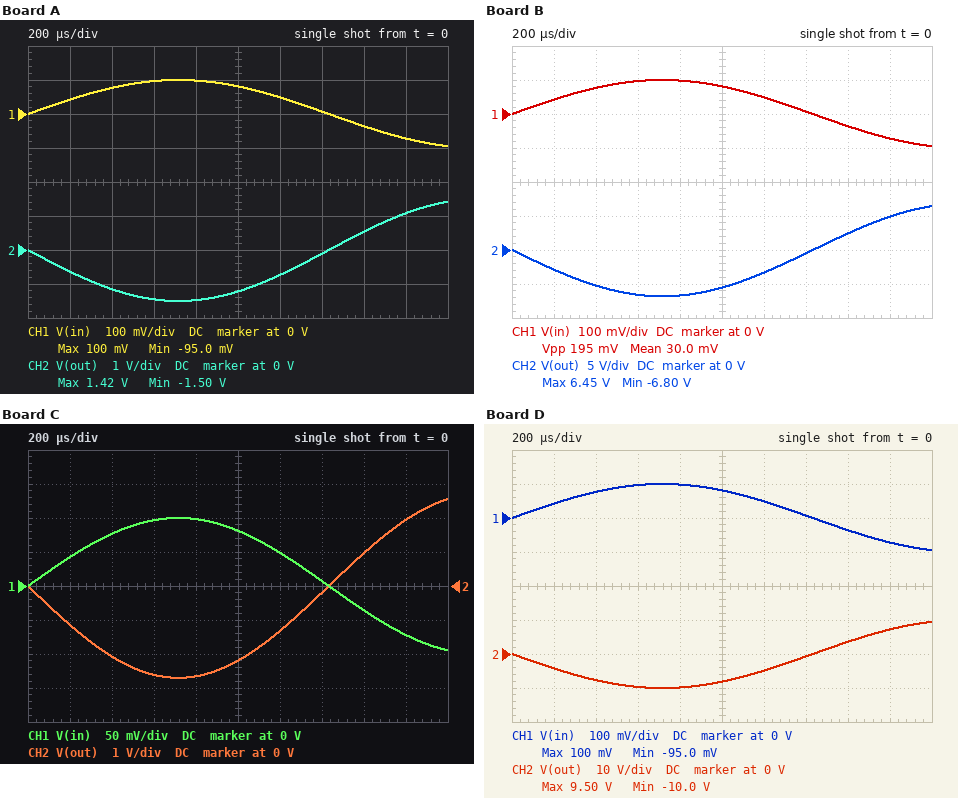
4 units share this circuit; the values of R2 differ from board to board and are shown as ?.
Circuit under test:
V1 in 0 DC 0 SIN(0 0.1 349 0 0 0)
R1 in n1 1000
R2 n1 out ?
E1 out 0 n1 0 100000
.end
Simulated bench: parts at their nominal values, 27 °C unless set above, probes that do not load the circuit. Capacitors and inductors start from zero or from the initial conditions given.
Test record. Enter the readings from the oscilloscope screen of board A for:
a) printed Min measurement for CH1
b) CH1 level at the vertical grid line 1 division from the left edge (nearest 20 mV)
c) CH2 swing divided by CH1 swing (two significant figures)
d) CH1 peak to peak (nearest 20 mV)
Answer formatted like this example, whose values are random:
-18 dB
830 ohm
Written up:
-95.0 mV
40 mV
15
200 mV
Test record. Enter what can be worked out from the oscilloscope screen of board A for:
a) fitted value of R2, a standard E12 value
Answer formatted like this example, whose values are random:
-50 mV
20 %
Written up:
15 kΩ
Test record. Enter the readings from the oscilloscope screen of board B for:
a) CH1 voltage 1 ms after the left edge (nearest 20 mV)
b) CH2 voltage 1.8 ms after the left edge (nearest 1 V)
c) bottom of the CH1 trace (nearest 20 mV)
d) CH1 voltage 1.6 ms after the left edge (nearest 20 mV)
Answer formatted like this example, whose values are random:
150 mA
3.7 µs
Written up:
80 mV
5 V
-100 mV
-40 mV
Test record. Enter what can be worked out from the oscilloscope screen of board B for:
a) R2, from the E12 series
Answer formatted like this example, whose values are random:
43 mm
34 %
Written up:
68 kΩ
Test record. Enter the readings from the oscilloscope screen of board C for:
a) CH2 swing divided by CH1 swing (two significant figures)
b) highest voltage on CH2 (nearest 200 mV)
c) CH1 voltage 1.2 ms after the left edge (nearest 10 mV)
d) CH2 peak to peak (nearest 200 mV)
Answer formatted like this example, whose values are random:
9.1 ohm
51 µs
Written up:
27
2.6 V
50 mV
5.2 V
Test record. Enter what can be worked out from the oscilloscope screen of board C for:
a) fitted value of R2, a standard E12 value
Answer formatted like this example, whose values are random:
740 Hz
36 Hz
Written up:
27 kΩ
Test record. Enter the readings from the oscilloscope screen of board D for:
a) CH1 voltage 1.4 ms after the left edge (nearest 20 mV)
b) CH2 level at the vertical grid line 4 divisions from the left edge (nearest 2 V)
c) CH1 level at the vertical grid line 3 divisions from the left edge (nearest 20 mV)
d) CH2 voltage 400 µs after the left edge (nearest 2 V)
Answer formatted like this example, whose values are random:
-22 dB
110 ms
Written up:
0 V
-10 V
100 mV
-8 V
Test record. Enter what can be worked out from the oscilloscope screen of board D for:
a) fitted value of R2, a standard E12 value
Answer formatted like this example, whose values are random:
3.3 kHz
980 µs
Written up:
100 kΩ
